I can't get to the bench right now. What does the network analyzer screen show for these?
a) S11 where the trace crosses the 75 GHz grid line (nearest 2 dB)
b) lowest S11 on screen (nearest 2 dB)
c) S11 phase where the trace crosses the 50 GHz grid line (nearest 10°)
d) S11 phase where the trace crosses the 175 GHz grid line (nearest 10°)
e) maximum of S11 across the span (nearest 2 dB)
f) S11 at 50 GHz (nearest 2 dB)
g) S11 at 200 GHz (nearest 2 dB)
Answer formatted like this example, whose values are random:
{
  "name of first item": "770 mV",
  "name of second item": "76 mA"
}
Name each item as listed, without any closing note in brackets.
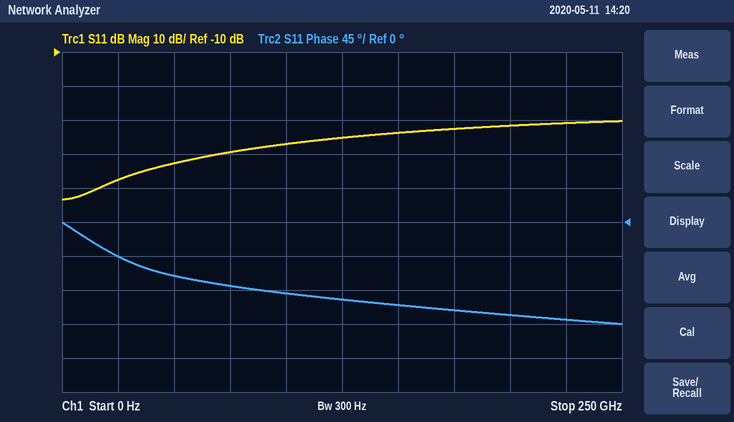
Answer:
{
  "S11 where the trace crosses the 75 GHz grid line": "-40 dB",
  "lowest S11 on screen": "-54 dB",
  "S11 phase where the trace crosses the 50 GHz grid line": "-70°",
  "S11 phase where the trace crosses the 175 GHz grid line": "-120°",
  "maximum of S11 across the span": "-30 dB",
  "S11 at 50 GHz": "-42 dB",
  "S11 at 200 GHz": "-32 dB"
}
